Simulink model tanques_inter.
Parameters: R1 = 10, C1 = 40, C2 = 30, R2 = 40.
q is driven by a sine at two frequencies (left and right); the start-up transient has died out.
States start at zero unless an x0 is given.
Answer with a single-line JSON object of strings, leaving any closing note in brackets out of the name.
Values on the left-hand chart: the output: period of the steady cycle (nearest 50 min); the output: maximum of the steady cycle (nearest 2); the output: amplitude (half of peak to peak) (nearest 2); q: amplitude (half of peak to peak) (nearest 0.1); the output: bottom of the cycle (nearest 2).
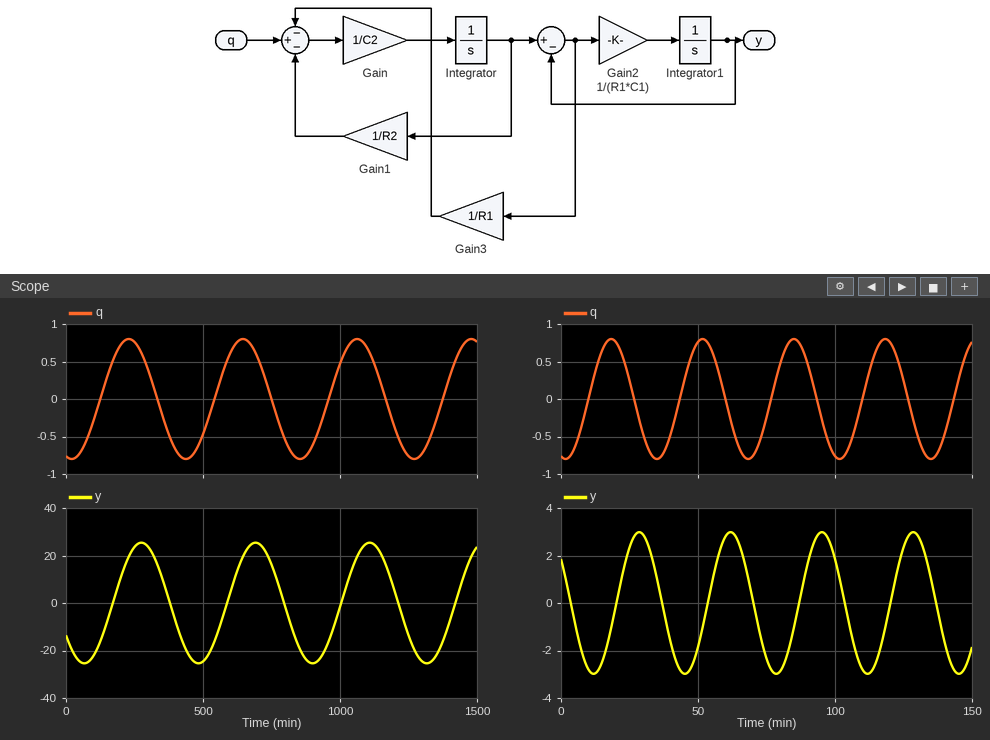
{"the output: period of the steady cycle": "400 min", "the output: maximum of the steady cycle": "26", "the output: amplitude (half of peak to peak)": "26", "q: amplitude (half of peak to peak)": "0.8", "the output: bottom of the cycle": "-26"}
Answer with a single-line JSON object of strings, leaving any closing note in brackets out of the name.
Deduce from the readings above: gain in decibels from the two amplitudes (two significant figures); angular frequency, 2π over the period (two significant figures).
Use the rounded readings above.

{"gain in decibels from the two amplitudes": "30 dB", "angular frequency, 2π over the period": "0.016 rad/min"}
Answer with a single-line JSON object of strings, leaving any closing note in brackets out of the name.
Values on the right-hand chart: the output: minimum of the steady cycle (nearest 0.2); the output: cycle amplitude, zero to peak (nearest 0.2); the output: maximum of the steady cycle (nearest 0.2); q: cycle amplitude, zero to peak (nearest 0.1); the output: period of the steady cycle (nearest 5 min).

{"the output: minimum of the steady cycle": "-3.0", "the output: cycle amplitude, zero to peak": "3.0", "the output: maximum of the steady cycle": "3.0", "q: cycle amplitude, zero to peak": "0.8", "the output: period of the steady cycle": "35 min"}
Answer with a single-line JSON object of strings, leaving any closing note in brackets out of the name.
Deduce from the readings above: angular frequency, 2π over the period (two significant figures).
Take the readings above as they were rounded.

{"angular frequency, 2π over the period": "0.18 rad/min"}
